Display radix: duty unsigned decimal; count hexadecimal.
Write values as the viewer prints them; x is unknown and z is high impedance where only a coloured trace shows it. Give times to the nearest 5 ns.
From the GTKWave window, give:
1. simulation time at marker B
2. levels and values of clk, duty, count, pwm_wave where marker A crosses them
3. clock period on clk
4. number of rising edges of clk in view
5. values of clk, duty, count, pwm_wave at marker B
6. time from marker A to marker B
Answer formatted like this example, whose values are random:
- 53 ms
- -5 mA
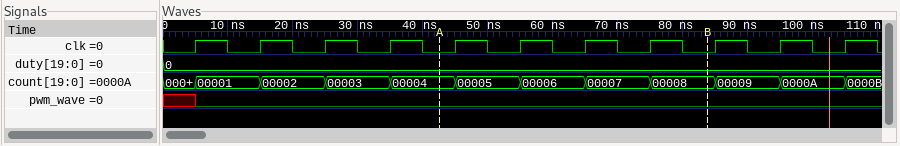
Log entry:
- 85 ns
- clk=0, duty=0, count=00004, pwm_wave=0
- 10 ns
- 11
- clk=0, duty=0, count=00008, pwm_wave=0
- 40 ns
